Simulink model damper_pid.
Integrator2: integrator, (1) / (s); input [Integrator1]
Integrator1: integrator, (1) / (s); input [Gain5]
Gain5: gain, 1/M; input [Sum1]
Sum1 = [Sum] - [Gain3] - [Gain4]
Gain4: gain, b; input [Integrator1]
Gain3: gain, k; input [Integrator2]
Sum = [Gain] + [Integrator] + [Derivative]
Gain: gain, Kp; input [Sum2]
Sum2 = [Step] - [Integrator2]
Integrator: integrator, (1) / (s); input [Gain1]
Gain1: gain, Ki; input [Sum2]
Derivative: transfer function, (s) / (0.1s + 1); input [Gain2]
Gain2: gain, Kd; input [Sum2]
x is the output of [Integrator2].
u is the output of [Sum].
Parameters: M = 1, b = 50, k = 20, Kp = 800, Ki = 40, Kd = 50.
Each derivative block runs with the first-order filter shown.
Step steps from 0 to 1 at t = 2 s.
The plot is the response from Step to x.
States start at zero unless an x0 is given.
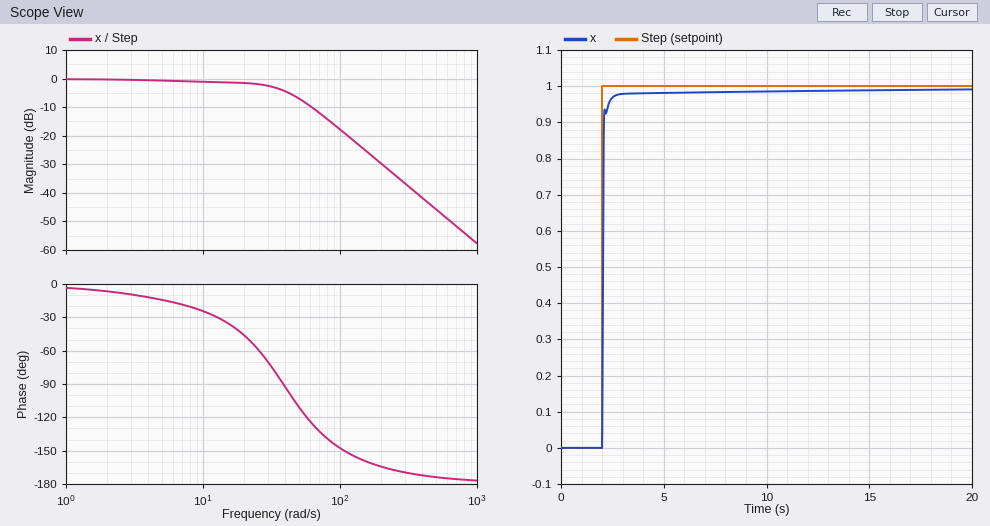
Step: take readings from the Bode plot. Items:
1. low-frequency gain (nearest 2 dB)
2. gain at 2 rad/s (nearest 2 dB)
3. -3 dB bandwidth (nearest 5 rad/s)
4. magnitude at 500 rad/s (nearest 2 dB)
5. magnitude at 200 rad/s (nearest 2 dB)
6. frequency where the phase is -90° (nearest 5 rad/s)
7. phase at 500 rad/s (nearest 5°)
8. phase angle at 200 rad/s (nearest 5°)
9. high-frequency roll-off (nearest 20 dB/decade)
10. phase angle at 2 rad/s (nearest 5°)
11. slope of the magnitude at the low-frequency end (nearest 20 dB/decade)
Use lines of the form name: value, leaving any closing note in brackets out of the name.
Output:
low-frequency gain: 0 dB
gain at 2 rad/s: 0 dB
-3 dB bandwidth: 35 rad/s
magnitude at 500 rad/s: -46 dB
magnitude at 200 rad/s: -30 dB
frequency where the phase is -90°: 40 rad/s
phase at 500 rad/s: -175°
phase angle at 200 rad/s: -165°
high-frequency roll-off: -40 dB/decade
phase angle at 2 rad/s: -5°
slope of the magnitude at the low-frequency end: 0 dB/decade
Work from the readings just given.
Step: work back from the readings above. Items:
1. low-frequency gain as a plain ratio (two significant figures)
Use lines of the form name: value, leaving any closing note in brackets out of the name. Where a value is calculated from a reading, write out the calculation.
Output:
low-frequency gain as a plain ratio: 10^(0 / 20) = 1.0
